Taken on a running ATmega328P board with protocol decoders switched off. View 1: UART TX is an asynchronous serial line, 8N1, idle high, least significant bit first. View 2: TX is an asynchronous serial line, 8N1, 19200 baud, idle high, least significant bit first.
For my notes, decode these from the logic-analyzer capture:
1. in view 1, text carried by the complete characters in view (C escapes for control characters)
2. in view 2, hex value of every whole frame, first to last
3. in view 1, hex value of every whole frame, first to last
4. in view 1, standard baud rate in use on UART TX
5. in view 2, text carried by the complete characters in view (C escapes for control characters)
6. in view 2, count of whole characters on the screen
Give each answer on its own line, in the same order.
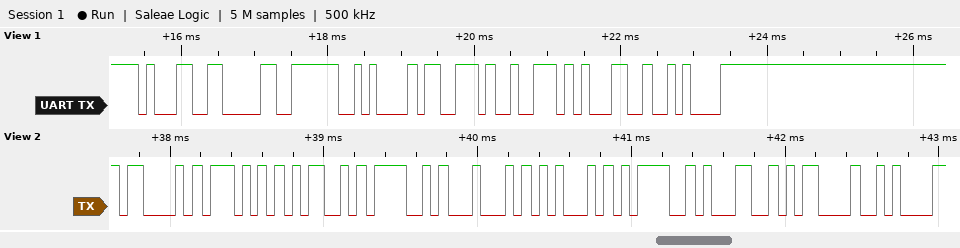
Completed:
"10\nsr1\n"
43 57 4D 4F 44 45 3D 31 0D 0A
0x31 0x30 0x0A 0x73 0x72 0x31 0x0A
9600 baud
"CWMODE=1\r\n"
10
